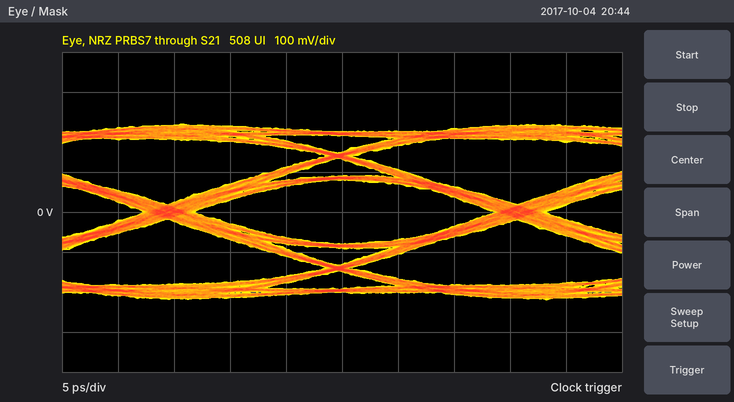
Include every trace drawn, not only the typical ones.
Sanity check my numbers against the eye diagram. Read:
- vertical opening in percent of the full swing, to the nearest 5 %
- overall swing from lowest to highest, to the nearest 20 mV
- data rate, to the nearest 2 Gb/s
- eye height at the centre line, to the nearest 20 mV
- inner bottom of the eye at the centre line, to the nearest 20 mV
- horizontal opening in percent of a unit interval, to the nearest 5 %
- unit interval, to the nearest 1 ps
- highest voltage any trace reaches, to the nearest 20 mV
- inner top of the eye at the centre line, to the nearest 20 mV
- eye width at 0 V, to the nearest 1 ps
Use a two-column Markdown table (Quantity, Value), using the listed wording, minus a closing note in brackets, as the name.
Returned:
| Quantity | Value |
|---|---|
| vertical opening in percent of the full swing, to the nearest 5 % | 35 % |
| overall swing from lowest to highest, to the nearest 20 mV | 440 mV |
| data rate, to the nearest 2 Gb/s | 32 Gb/s |
| eye height at the centre line, to the nearest 20 mV | 160 mV |
| inner bottom of the eye at the centre line, to the nearest 20 mV | -80 mV |
| horizontal opening in percent of a unit interval, to the nearest 5 % | 85 % |
| unit interval, to the nearest 1 ps | 31 ps |
| highest voltage any trace reaches, to the nearest 20 mV | 220 mV |
| inner top of the eye at the centre line, to the nearest 20 mV | 80 mV |
| eye width at 0 V, to the nearest 1 ps | 27 ps |
